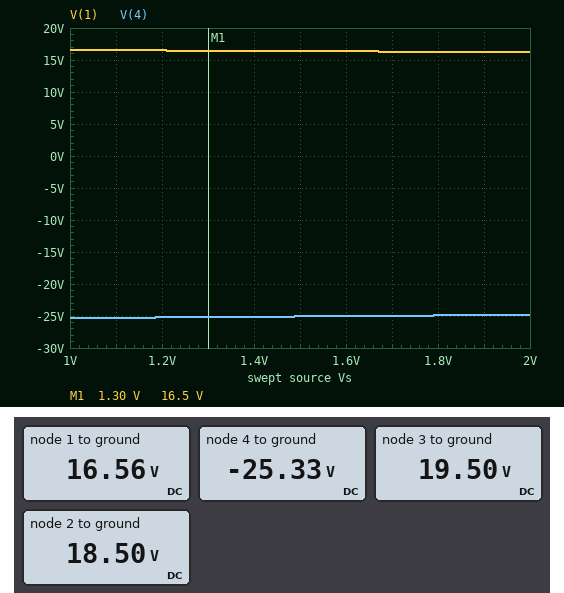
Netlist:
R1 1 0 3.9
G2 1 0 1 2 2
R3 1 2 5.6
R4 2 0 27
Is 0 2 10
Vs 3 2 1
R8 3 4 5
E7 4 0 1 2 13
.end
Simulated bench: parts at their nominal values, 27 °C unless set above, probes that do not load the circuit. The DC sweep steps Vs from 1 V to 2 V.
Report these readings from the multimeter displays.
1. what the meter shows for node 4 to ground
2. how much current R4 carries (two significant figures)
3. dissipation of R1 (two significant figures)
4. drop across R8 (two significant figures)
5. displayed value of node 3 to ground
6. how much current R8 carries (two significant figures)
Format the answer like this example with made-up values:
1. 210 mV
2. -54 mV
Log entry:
1. -25.33 V
2. 690 mA
3. 70 W
4. 45 V
5. 19.50 V
6. 9.0 A
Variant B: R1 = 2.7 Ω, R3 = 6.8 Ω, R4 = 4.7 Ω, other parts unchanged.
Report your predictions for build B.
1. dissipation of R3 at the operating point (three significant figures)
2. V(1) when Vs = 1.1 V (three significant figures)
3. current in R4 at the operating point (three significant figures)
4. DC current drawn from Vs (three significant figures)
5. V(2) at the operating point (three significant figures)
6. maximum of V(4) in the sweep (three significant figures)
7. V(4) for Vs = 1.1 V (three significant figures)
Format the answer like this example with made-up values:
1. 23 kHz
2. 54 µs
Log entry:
1. 458 mW
2. 10.2 V
3. 2.55 A
4. 7.19 A
5. 12.0 V
6. -22.5 V
7. -22.9 V
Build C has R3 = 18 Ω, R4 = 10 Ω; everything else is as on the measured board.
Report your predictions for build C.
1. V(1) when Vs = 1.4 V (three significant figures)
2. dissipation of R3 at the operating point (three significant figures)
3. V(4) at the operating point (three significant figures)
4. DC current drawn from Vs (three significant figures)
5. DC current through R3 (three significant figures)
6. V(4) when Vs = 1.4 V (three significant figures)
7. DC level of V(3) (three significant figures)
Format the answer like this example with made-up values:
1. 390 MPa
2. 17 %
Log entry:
1. 14.5 V
2. 186 mW
3. -23.8 V
4. 8.25 A
5. 102 mA
6. -23.6 V
7. 17.5 V
